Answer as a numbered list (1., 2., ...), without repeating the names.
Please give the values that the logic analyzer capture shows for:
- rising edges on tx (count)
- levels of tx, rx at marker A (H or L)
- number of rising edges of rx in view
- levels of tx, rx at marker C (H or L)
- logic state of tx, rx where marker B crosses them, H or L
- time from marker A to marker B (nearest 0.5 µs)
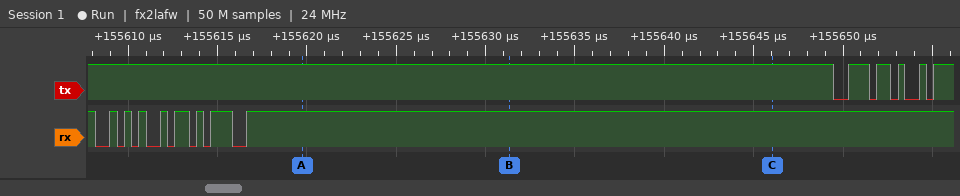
1. 5
2. tx=H, rx=H
3. 8
4. tx=H, rx=H
5. tx=H, rx=H
6. 11.5 µs
